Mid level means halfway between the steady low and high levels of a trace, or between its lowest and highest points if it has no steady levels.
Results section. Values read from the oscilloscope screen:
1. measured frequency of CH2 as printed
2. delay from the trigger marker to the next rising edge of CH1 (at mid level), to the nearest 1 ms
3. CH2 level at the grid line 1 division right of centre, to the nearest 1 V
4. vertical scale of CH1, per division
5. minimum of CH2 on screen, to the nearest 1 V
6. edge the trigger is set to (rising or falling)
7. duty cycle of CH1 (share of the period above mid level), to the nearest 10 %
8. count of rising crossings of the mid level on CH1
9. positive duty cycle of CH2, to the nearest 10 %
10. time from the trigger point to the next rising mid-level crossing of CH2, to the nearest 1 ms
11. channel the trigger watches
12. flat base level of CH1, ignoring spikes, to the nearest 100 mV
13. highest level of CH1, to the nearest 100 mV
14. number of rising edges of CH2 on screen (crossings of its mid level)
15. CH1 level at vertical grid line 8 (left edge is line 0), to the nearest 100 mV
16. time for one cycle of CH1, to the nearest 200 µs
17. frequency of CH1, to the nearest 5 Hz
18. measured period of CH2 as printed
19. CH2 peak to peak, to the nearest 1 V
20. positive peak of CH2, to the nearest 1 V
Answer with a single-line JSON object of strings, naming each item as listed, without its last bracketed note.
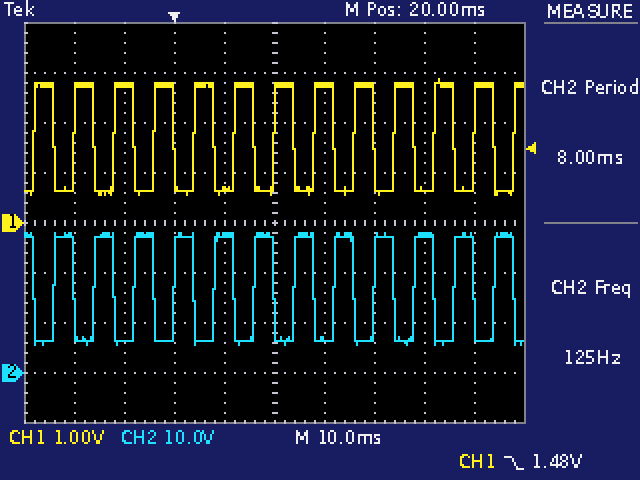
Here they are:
{"measured frequency of CH2 as printed": "125 Hz", "delay from the trigger marker to the next rising edge of CH1 (at mid level), to the nearest 1 ms": "4 ms", "CH2 level at the grid line 1 division right of centre, to the nearest 1 V": "7 V", "vertical scale of CH1, per division": "1 V", "minimum of CH2 on screen, to the nearest 1 V": "6 V", "edge the trigger is set to": "falling", "duty cycle of CH1 (share of the period above mid level), to the nearest 10 %": "50 %", "count of rising crossings of the mid level on CH1": "13", "positive duty cycle of CH2, to the nearest 10 %": "50 %", "time from the trigger point to the next rising mid-level crossing of CH2, to the nearest 1 ms": "8 ms", "channel the trigger watches": "CH1", "flat base level of CH1, ignoring spikes, to the nearest 100 mV": "600 mV", "highest level of CH1, to the nearest 100 mV": "2.9 V", "number of rising edges of CH2 on screen": "12", "CH1 level at vertical grid line 8 (left edge is line 0), to the nearest 100 mV": "700 mV", "time for one cycle of CH1, to the nearest 200 µs": "8.0 ms", "frequency of CH1, to the nearest 5 Hz": "125 Hz", "measured period of CH2 as printed": "8.00 ms", "CH2 peak to peak, to the nearest 1 V": "22 V", "positive peak of CH2, to the nearest 1 V": "28 V"}
